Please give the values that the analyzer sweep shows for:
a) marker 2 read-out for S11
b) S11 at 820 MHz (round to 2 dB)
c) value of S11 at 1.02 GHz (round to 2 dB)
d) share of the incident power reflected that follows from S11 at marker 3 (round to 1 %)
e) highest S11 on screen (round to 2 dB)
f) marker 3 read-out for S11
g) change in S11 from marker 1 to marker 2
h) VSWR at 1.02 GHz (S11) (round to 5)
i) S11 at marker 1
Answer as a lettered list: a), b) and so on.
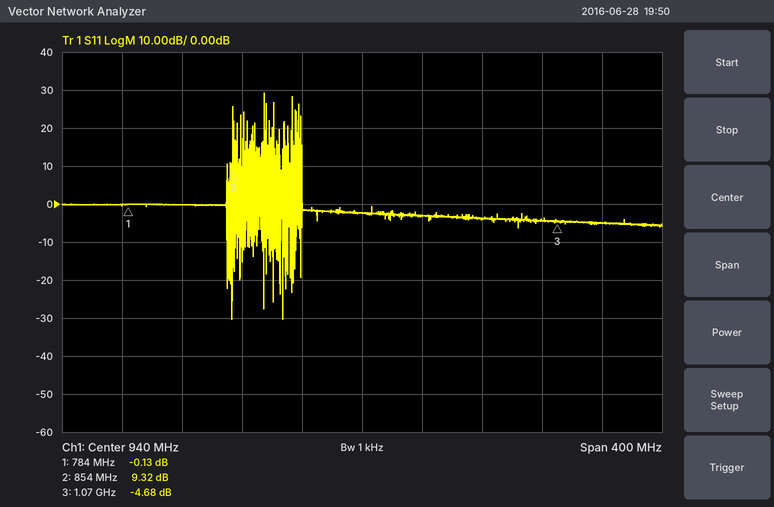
a) 9.32 dB
b) 0 dB
c) -4 dB
d) 34 %
e) 30 dB
f) -4.68 dB
g) 9.45 dB
h) 5
i) -0.13 dB
